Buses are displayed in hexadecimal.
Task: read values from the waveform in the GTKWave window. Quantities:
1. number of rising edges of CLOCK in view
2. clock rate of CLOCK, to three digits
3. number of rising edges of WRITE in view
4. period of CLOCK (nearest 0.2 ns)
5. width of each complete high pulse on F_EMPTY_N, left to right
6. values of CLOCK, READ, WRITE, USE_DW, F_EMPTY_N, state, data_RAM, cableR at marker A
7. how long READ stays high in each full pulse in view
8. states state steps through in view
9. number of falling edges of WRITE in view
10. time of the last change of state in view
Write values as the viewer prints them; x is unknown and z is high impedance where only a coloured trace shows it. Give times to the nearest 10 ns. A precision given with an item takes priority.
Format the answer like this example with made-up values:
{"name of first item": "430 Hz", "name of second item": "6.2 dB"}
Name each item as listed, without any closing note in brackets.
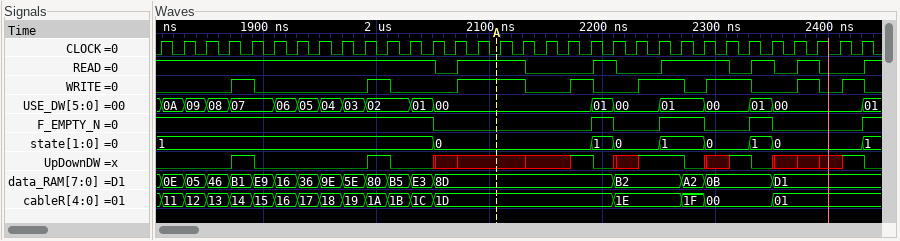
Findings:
{"number of rising edges of CLOCK in view": "32", "clock rate of CLOCK, to three digits": "50.0 MHz", "number of rising edges of WRITE in view": "8", "period of CLOCK": "20 ns", "width of each complete high pulse on F_EMPTY_N, left to right": "20 ns, 40 ns, 20 ns", "values of CLOCK, READ, WRITE, USE_DW, F_EMPTY_N, state, data_RAM, cableR at marker A": "CLOCK=0, READ=1, WRITE=1, USE_DW=00, F_EMPTY_N=0, state=0, data_RAM=8D, cableR=1D", "how long READ stays high in each full pulse in view": "60 ns, 20 ns, 60 ns, 20 ns, 20 ns", "states state steps through in view": "1, 0, 1, 0, 1, 0, 1, 0, 1", "number of falling edges of WRITE in view": "8", "time of the last change of state in view": "2430 ns"}
